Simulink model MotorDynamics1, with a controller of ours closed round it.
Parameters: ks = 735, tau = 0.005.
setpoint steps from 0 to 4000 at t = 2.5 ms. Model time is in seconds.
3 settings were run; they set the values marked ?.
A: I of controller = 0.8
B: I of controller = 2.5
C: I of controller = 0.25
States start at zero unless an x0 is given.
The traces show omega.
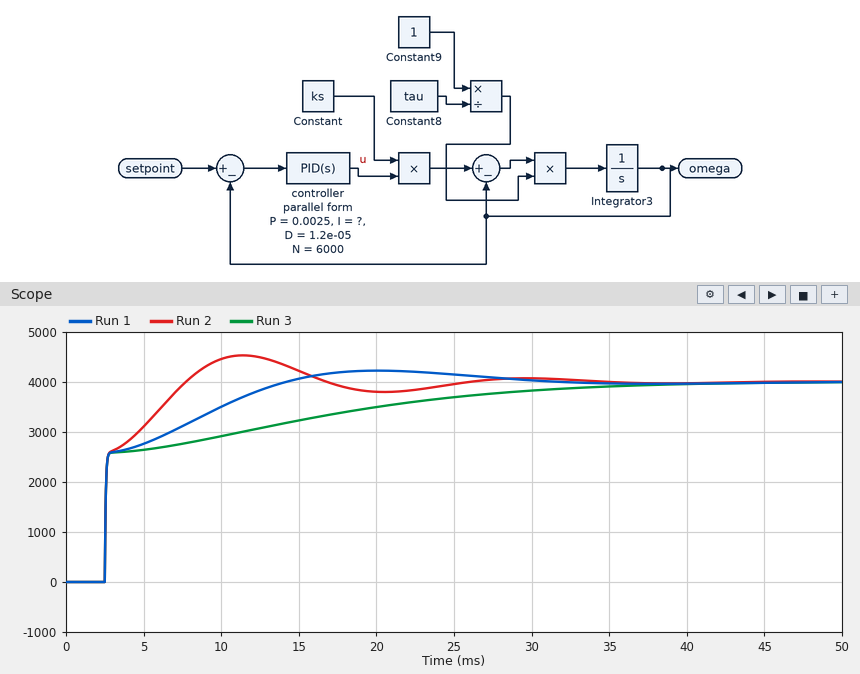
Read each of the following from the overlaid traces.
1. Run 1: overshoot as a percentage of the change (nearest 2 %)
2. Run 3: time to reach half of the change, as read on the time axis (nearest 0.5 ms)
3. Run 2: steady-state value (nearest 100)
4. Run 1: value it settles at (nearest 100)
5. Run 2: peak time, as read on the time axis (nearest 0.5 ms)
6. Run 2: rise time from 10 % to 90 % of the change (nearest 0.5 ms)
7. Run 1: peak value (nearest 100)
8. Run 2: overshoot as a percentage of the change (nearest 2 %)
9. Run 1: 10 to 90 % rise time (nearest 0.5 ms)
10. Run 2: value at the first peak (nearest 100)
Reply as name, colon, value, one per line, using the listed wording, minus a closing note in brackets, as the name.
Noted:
Run 1: overshoot as a percentage of the change: 6 %
Run 3: time to reach half of the change, as read on the time axis: 2.5 ms
Run 2: steady-state value: 4000
Run 1: value it settles at: 4000
Run 2: peak time, as read on the time axis: 11.5 ms
Run 2: rise time from 10 % to 90 % of the change: 4.0 ms
Run 1: peak value: 4200
Run 2: overshoot as a percentage of the change: 14 %
Run 1: 10 to 90 % rise time: 8.0 ms
Run 2: value at the first peak: 4500
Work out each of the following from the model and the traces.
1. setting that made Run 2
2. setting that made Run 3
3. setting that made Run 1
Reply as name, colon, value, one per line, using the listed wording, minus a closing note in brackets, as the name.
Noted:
setting that made Run 2: B
setting that made Run 3: C
setting that made Run 1: A
